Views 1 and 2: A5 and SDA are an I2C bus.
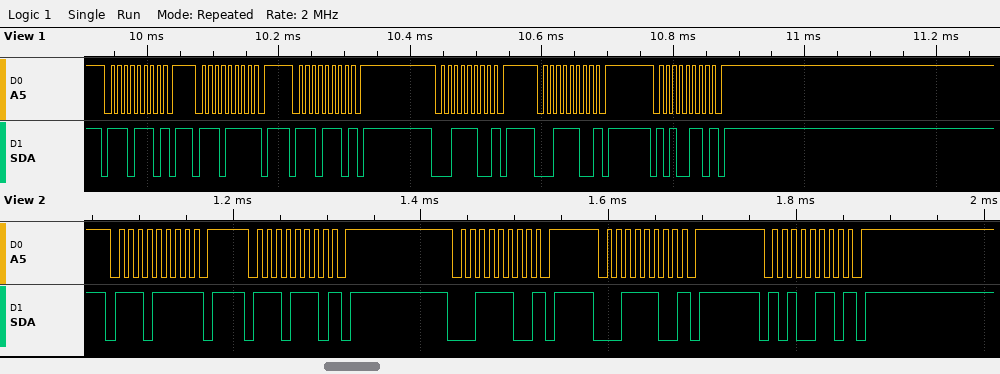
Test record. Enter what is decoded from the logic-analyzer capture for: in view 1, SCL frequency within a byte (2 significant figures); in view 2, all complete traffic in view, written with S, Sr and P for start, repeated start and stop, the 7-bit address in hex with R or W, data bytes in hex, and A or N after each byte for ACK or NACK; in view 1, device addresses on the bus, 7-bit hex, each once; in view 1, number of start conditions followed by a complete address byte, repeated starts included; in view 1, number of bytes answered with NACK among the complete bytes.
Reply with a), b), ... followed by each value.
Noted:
a) 100 kHz
b) S 77R N P S 77W N P S 1EW N P S 1EW N P S 53W N P
c) 0x77 0x1E 0x53
d) 6
e) 6
